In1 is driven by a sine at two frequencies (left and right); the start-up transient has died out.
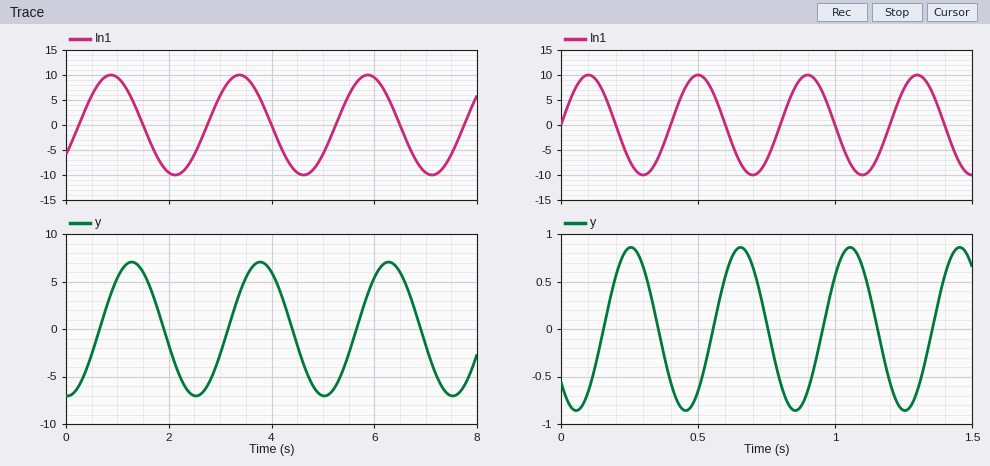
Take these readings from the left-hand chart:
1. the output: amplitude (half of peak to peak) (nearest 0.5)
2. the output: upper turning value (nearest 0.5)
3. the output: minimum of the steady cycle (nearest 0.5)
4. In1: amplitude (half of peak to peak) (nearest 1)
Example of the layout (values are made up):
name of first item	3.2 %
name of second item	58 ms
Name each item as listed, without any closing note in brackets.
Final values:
the output: amplitude (half of peak to peak)	7.0
the output: upper turning value	7.0
the output: minimum of the steady cycle	-7.0
In1: amplitude (half of peak to peak)	10
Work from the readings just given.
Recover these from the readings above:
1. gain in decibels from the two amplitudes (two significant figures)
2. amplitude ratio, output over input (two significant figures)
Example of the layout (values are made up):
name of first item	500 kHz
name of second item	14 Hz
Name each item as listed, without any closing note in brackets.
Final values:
gain in decibels from the two amplitudes	-3.1 dB
amplitude ratio, output over input	0.70
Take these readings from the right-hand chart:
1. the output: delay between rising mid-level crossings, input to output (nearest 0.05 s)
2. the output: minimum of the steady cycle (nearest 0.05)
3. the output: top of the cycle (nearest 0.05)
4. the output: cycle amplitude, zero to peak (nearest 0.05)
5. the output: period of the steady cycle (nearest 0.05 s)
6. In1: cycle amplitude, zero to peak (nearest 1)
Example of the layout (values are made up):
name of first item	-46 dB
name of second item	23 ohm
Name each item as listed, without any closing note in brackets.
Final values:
the output: delay between rising mid-level crossings, input to output	0.15 s
the output: minimum of the steady cycle	-0.85
the output: top of the cycle	0.85
the output: cycle amplitude, zero to peak	0.85
the output: period of the steady cycle	0.40 s
In1: cycle amplitude, zero to peak	10
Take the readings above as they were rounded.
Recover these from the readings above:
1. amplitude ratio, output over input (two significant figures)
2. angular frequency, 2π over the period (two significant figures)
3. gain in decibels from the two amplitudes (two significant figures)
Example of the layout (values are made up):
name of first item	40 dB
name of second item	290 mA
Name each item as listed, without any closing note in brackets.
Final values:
amplitude ratio, output over input	0.085
angular frequency, 2π over the period	16 rad/s
gain in decibels from the two amplitudes	-21 dB
